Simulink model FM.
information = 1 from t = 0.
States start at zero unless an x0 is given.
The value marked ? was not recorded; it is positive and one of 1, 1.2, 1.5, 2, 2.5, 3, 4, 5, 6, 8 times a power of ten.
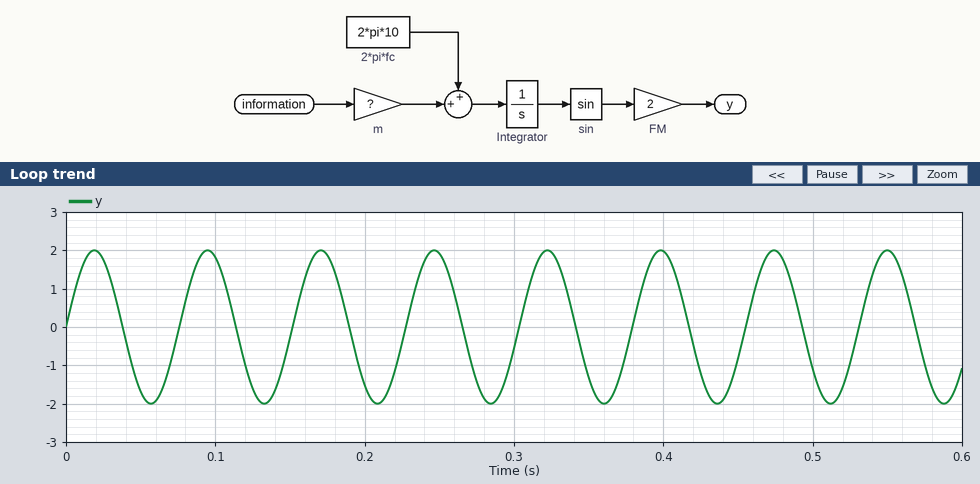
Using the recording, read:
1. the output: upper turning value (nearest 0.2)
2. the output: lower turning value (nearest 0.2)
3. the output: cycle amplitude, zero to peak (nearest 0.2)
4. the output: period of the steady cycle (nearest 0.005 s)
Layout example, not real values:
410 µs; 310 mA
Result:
2.0; -2.0; 2.0; 0.075 s
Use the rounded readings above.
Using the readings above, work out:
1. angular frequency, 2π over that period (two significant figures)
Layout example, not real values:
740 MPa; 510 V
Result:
84 rad/s
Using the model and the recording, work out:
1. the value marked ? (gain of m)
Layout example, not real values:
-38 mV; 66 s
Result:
20
